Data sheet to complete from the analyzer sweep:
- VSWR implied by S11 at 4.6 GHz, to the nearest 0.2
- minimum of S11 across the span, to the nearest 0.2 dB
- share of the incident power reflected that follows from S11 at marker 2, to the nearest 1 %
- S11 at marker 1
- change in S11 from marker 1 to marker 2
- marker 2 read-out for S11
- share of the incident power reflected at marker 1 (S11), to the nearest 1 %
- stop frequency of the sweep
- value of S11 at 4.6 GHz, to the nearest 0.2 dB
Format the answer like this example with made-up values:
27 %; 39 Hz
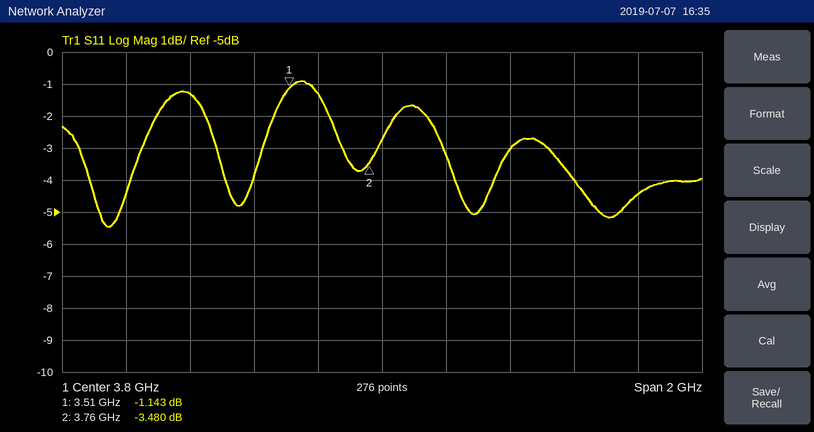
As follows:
4.0; -5.4 dB; 45 %; -1.143 dB; -2.337 dB; -3.480 dB; 77 %; 4.8 GHz; -4.4 dB
